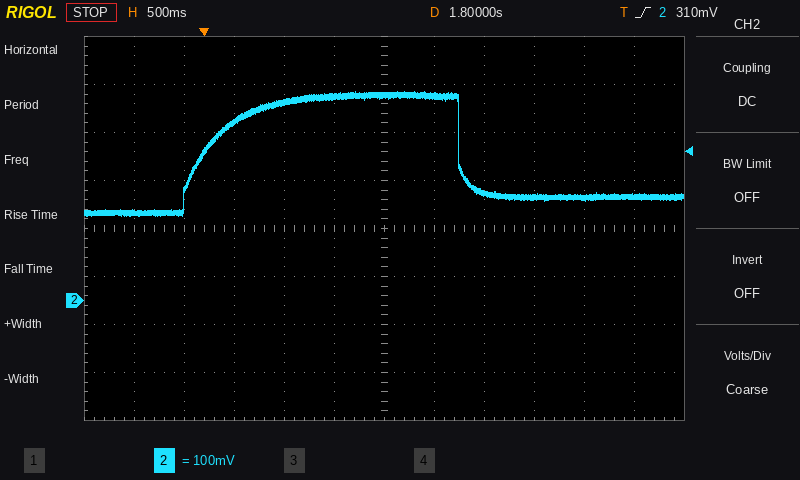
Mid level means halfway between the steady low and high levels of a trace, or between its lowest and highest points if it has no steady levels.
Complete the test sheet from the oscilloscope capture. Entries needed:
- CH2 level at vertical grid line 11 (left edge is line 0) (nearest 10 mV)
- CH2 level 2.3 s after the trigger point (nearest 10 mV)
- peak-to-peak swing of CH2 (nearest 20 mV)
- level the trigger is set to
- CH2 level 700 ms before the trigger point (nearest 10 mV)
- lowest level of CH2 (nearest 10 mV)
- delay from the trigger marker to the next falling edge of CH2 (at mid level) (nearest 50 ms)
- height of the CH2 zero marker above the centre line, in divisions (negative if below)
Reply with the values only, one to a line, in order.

220 mV
430 mV
260 mV
310 mV
180 mV
180 mV
2.55 s
-1.5 div
